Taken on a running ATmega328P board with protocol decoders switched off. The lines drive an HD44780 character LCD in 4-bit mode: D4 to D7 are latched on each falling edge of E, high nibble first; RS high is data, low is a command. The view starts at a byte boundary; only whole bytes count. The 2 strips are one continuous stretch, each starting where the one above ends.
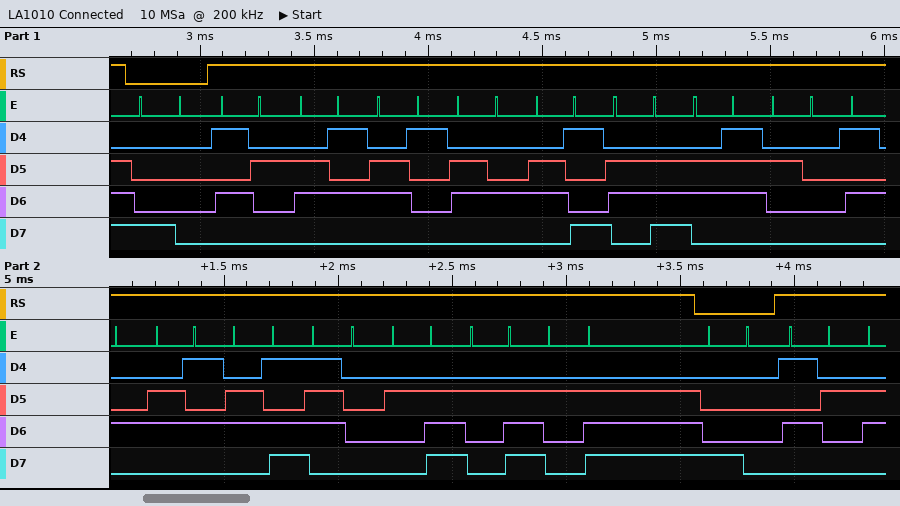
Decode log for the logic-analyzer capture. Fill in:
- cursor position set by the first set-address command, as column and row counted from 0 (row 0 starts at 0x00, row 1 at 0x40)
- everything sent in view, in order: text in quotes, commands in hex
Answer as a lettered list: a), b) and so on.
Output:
a) column 0, row 0
b) 0x80 "Reading Temp..." 0x80 "R"
